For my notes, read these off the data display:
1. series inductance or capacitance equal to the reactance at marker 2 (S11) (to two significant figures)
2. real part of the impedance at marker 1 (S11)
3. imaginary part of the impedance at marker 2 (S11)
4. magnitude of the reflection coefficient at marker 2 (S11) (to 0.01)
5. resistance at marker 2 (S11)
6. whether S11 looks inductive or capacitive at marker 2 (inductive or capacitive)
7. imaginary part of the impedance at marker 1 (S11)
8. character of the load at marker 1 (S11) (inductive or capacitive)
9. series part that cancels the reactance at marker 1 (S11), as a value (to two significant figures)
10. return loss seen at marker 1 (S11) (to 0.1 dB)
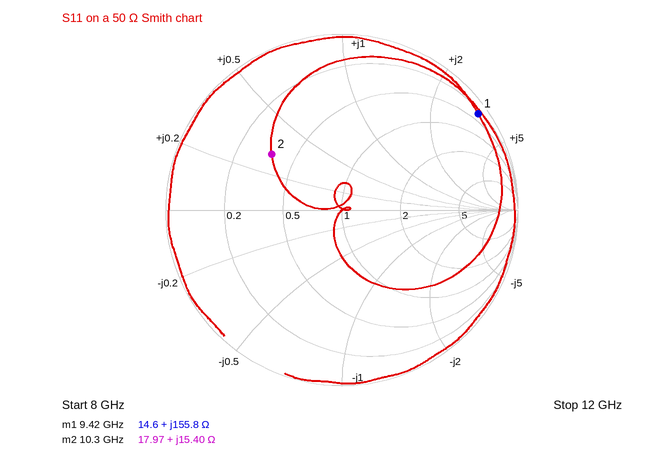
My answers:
240 pH
14.6 Ω
+15.40 Ω
0.51
17.97 Ω
inductive
+155.8 Ω
inductive
110 fF
0.5 dB
